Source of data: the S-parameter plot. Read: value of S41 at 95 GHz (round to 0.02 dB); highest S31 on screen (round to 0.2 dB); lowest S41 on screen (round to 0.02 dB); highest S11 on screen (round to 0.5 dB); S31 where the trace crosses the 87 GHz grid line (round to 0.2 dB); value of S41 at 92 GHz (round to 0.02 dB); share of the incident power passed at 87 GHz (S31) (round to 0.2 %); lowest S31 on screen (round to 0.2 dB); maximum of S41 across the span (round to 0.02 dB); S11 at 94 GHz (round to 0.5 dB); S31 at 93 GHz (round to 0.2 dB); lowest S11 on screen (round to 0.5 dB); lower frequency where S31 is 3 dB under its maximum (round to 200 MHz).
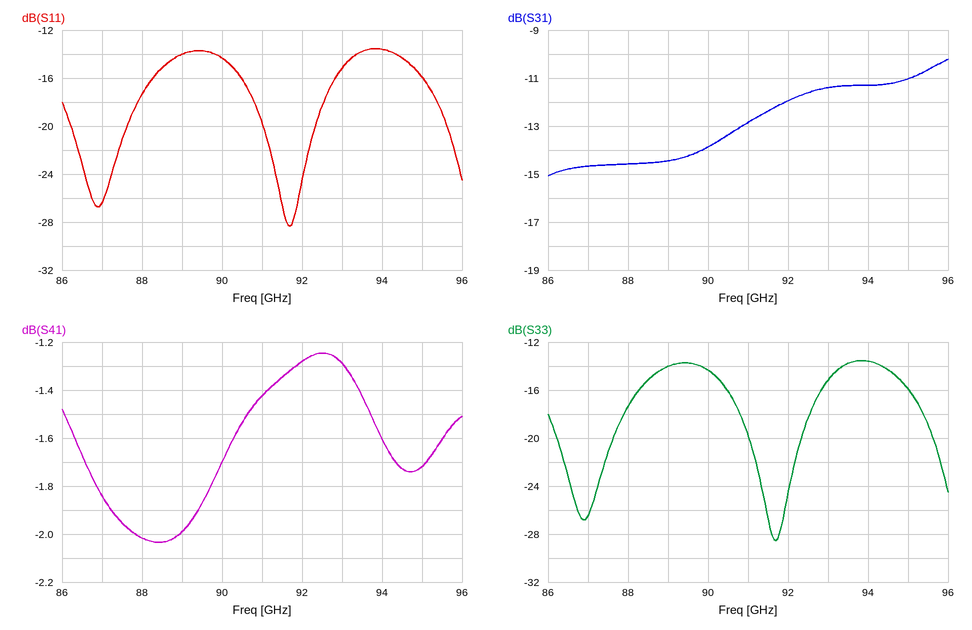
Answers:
-1.72 dB
-10.2 dB
-2.04 dB
-13.5 dB
-14.6 dB
-1.28 dB
3.4 %
-15.0 dB
-1.24 dB
-13.5 dB
-11.4 dB
-28.5 dB
90.6 GHz
